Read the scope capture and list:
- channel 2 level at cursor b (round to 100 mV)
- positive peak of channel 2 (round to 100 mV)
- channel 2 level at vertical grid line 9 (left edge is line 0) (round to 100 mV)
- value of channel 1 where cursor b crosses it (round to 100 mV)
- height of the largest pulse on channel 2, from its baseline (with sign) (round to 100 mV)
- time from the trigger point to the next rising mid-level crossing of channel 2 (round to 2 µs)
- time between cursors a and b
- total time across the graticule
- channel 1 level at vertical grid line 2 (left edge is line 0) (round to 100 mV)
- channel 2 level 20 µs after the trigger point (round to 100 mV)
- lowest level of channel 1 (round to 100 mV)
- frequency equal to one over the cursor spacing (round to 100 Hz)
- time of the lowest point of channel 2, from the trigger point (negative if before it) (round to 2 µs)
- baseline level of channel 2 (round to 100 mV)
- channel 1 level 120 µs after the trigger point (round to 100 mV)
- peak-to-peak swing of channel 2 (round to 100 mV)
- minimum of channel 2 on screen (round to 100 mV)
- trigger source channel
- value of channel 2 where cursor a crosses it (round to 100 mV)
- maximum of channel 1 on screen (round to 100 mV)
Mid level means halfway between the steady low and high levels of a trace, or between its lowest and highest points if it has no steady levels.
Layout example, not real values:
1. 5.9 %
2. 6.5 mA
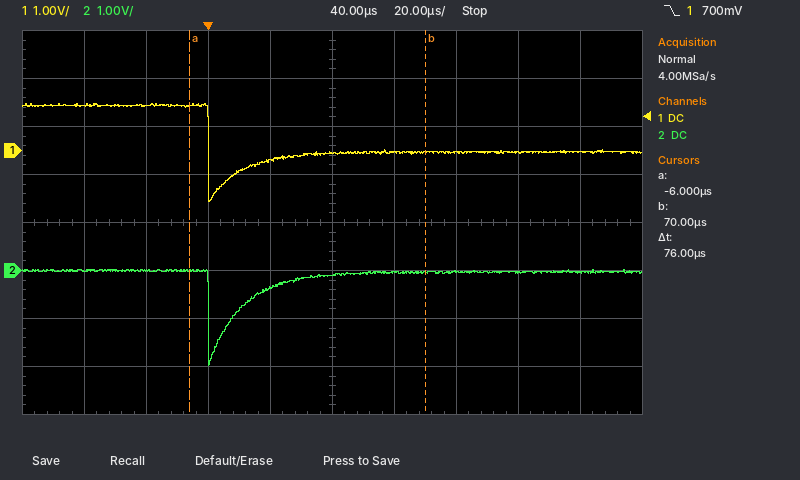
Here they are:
1. 0.0 V
2. 0.0 V
3. 0.0 V
4. 0.0 V
5. -2.0 V
6. 8 µs
7. 76 µs
8. 200 µs
9. 900 mV
10. -400 mV
11. -1.1 V
12. 13.2 kHz
13. 0 µs
14. 0.0 V
15. 0.0 V
16. 2.0 V
17. -2.0 V
18. channel 1
19. 0.0 V
20. 1.0 V
